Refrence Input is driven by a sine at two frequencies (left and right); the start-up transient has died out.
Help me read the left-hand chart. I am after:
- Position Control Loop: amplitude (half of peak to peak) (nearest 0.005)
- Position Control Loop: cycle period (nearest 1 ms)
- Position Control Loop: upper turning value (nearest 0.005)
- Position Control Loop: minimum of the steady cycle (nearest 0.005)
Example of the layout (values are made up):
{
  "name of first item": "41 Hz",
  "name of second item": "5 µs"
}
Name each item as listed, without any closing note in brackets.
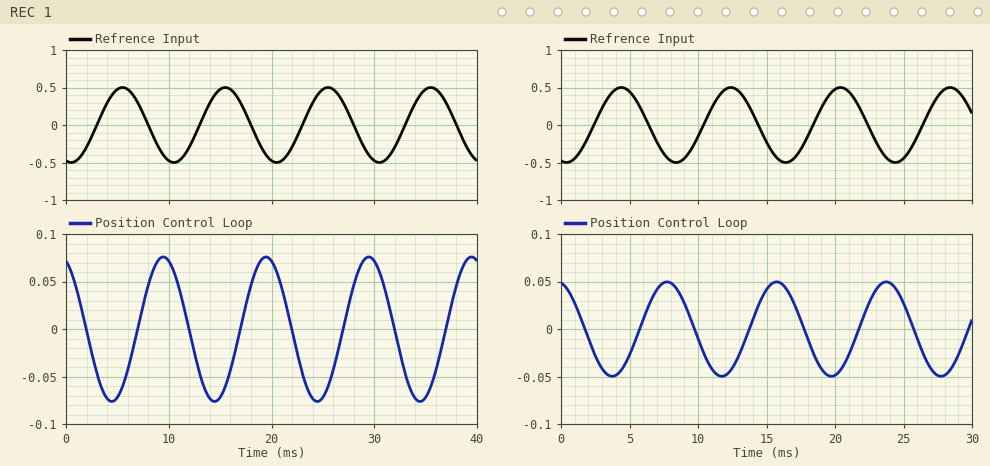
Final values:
{
  "Position Control Loop: amplitude (half of peak to peak)": "0.075",
  "Position Control Loop: cycle period": "10 ms",
  "Position Control Loop: upper turning value": "0.075",
  "Position Control Loop: minimum of the steady cycle": "-0.075"
}
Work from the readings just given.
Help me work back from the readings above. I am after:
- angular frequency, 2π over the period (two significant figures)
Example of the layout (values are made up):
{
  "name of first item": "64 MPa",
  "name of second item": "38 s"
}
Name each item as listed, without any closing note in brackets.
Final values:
{
  "angular frequency, 2π over the period": "0.63 rad/ms"
}
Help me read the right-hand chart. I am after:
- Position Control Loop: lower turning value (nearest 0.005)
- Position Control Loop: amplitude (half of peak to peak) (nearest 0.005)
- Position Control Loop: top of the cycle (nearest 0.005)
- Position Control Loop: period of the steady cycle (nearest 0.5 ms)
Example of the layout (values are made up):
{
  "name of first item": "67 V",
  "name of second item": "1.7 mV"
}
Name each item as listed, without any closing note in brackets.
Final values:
{
  "Position Control Loop: lower turning value": "-0.050",
  "Position Control Loop: amplitude (half of peak to peak)": "0.050",
  "Position Control Loop: top of the cycle": "0.050",
  "Position Control Loop: period of the steady cycle": "8.0 ms"
}
